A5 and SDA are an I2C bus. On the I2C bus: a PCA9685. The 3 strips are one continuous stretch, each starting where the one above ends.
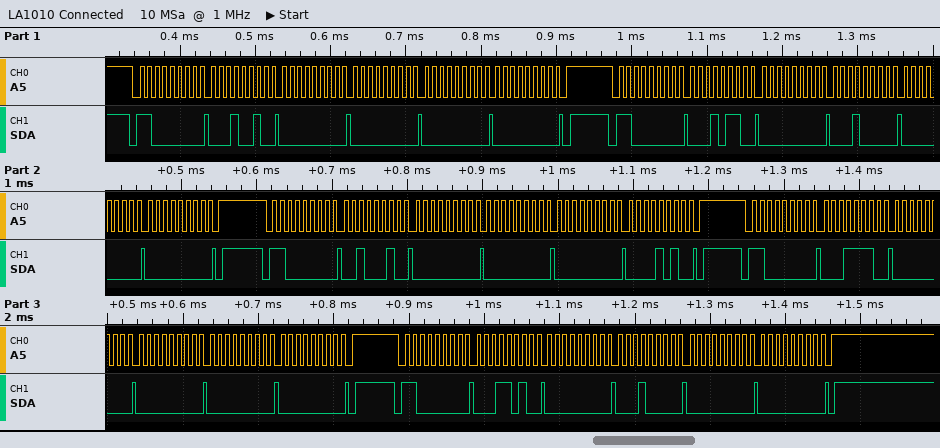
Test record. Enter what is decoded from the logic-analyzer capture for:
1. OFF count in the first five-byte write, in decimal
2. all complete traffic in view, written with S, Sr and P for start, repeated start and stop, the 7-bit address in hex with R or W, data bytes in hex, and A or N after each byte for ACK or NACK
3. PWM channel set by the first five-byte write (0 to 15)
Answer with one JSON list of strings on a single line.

["0", "S 60W A 12 A 00 A 00 A 00 A 00 A P S 60W A 16 A 00 A 10 A 00 A 00 A P S 60W A 22 A 00 A 00 A 00 A 0A A P S 60W A 1E A 00 A 00 A 00 A 00 A P S 60W A 1A A 00 A 10 A 00 A 00 A P", "3"]
